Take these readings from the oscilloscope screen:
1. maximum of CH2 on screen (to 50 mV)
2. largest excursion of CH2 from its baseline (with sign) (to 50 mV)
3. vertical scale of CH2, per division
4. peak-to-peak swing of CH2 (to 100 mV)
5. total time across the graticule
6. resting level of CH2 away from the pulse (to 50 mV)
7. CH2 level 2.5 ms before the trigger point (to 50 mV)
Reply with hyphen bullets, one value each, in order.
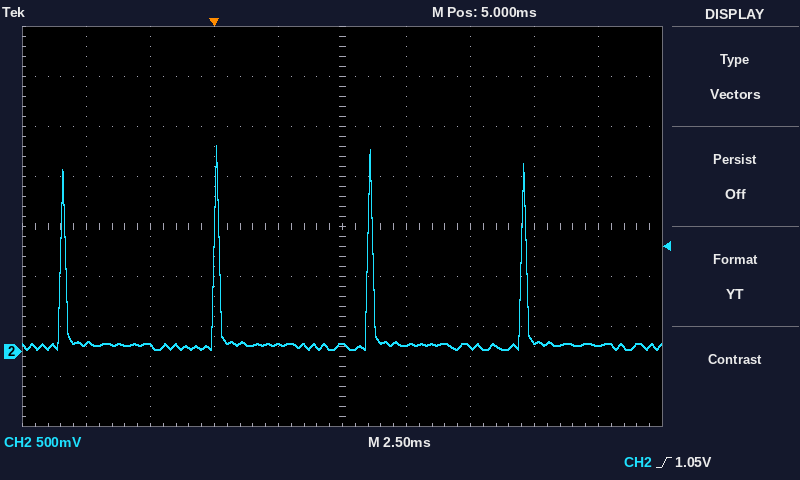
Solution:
- 2.05 V
- +2.00 V
- 500 mV
- 2.00 V
- 25 ms
- 50 mV
- 50 mV
